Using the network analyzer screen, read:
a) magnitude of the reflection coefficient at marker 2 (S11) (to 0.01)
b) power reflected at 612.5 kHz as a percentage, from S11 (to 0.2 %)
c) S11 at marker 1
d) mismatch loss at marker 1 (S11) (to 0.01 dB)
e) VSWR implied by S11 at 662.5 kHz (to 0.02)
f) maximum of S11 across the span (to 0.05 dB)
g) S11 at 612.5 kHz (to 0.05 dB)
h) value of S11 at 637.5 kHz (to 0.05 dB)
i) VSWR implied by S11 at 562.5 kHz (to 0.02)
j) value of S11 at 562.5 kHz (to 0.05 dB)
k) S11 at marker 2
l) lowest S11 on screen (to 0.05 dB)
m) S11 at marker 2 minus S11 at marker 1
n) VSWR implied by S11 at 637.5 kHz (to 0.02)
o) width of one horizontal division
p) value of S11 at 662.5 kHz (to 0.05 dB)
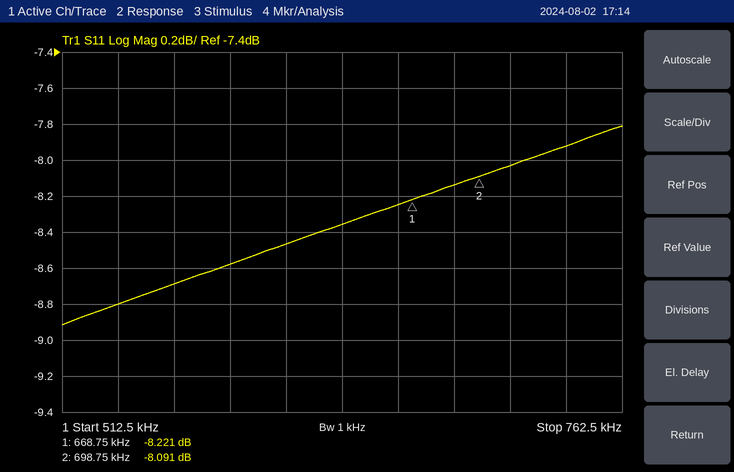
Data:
0.39
14.2 %
-8.221 dB
0.71 dB
2.26
-7.80 dB
-8.45 dB
-8.35 dB
2.16
-8.70 dB
-8.091 dB
-8.90 dB
0.130 dB
2.24
25 kHz
-8.25 dB
